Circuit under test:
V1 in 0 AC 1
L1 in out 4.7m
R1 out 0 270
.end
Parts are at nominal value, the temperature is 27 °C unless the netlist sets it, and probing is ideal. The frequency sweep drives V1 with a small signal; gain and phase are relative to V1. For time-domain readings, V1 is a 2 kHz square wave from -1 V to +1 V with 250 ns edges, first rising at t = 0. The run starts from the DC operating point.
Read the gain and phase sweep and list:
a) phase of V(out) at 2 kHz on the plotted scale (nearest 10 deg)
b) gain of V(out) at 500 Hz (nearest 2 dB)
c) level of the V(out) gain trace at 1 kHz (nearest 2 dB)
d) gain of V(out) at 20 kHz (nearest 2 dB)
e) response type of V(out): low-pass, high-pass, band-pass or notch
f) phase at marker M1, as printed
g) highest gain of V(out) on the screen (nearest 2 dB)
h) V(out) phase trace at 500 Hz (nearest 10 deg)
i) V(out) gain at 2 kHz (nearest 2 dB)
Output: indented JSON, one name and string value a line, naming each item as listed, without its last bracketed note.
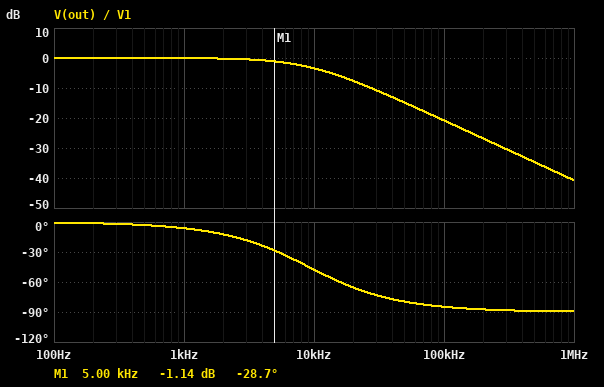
{
  "phase of V(out) at 2 kHz on the plotted scale": "-10 deg",
  "gain of V(out) at 500 Hz": "0 dB",
  "level of the V(out) gain trace at 1 kHz": "0 dB",
  "gain of V(out) at 20 kHz": "-8 dB",
  "response type of V(out): low-pass, high-pass, band-pass or notch": "low-pass",
  "phase at marker M1, as printed": "-28.7 deg",
  "highest gain of V(out) on the screen": "0 dB",
  "V(out) phase trace at 500 Hz": "0 deg",
  "V(out) gain at 2 kHz": "0 dB"
}
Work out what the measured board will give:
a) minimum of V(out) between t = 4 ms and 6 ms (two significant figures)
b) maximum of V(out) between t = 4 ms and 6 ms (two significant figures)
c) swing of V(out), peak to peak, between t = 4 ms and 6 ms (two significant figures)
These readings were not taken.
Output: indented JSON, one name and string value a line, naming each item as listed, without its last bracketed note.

{
  "minimum of V(out) between t = 4 ms and 6 ms": "-1.0 V",
  "maximum of V(out) between t = 4 ms and 6 ms": "1.0 V",
  "swing of V(out), peak to peak, between t = 4 ms and 6 ms": "2.0 V"
}
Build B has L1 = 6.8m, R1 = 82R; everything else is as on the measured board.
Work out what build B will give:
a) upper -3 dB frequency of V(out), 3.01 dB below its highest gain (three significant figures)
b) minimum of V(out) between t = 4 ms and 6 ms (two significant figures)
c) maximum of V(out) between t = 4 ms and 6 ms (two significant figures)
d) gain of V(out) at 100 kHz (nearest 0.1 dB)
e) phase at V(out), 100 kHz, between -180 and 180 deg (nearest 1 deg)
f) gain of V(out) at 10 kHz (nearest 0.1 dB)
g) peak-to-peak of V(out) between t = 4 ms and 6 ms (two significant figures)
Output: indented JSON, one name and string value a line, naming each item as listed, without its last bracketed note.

{
  "upper -3 dB frequency of V(out), 3.01 dB below its highest gain": "1.92 kHz",
  "minimum of V(out) between t = 4 ms and 6 ms": "-910 mV",
  "maximum of V(out) between t = 4 ms and 6 ms": "910 mV",
  "gain of V(out) at 100 kHz": "-34.3 dB",
  "phase at V(out), 100 kHz, between -180 and 180 deg": "-89 deg",
  "gain of V(out) at 10 kHz": "-14.5 dB",
  "peak-to-peak of V(out) between t = 4 ms and 6 ms": "1.8 V"
}
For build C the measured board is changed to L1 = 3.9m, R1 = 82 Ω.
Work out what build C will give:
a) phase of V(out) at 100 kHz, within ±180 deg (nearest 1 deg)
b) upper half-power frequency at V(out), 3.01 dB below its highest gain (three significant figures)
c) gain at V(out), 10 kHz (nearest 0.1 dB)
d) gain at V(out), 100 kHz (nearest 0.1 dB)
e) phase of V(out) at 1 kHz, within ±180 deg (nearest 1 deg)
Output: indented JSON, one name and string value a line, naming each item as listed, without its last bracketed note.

{
  "phase of V(out) at 100 kHz, within ±180 deg": "-88 deg",
  "upper half-power frequency at V(out), 3.01 dB below its highest gain": "3.35 kHz",
  "gain at V(out), 10 kHz": "-10.0 dB",
  "gain at V(out), 100 kHz": "-29.5 dB",
  "phase of V(out) at 1 kHz, within ±180 deg": "-17 deg"
}
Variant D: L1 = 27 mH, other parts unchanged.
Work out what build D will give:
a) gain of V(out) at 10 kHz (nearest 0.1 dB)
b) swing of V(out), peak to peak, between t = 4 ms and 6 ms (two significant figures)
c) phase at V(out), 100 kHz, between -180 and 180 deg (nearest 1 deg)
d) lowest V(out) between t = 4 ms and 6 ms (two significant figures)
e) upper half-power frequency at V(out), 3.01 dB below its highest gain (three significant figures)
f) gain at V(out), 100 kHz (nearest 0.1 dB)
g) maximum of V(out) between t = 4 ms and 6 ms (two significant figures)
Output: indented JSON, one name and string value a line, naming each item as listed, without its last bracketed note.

{
  "gain of V(out) at 10 kHz": "-16.1 dB",
  "swing of V(out), peak to peak, between t = 4 ms and 6 ms": "1.7 V",
  "phase at V(out), 100 kHz, between -180 and 180 deg": "-89 deg",
  "lowest V(out) between t = 4 ms and 6 ms": "-850 mV",
  "upper half-power frequency at V(out), 3.01 dB below its highest gain": "1.59 kHz",
  "gain at V(out), 100 kHz": "-36.0 dB",
  "maximum of V(out) between t = 4 ms and 6 ms": "850 mV"
}
